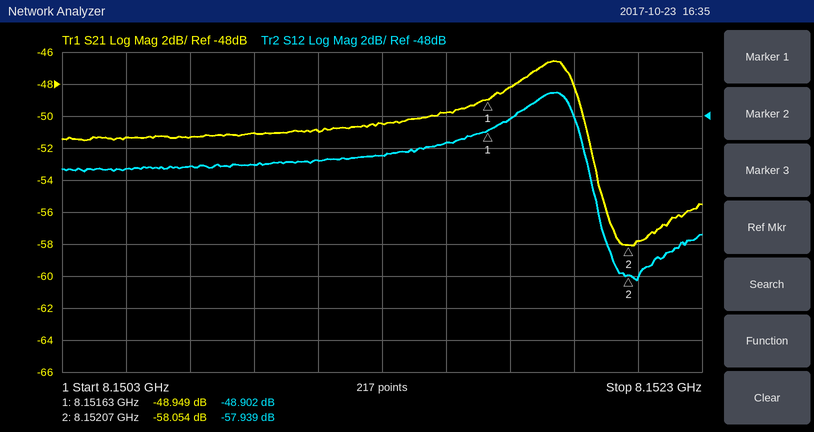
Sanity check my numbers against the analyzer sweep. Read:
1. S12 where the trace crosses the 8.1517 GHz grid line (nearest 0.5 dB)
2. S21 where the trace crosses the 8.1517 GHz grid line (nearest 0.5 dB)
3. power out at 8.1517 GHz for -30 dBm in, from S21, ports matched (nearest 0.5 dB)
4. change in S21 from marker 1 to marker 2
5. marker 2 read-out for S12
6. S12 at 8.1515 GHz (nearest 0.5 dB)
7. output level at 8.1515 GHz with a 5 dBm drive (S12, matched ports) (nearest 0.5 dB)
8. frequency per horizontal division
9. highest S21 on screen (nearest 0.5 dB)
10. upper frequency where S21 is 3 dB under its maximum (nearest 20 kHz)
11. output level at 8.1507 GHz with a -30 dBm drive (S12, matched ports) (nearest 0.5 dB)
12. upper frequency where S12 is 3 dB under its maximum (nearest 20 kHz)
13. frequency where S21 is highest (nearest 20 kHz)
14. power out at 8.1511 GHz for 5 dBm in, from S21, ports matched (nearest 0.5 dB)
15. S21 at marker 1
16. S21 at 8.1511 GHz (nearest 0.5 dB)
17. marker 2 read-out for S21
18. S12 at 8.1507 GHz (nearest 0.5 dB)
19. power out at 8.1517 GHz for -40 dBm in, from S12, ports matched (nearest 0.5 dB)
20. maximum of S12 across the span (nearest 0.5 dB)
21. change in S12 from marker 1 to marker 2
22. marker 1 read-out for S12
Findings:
-48.0 dB
-48.0 dB
-78.0 dBm
-9.105 dB
-57.939 dB
-49.5 dB
-44.5 dBm
200 kHz
-46.5 dB
8.15192 GHz
-81.0 dBm
8.15192 GHz
8.15184 GHz
-46.0 dBm
-48.949 dB
-51.0 dB
-58.054 dB
-51.0 dB
-88.0 dBm
-46.5 dB
-9.037 dB
-48.902 dB
